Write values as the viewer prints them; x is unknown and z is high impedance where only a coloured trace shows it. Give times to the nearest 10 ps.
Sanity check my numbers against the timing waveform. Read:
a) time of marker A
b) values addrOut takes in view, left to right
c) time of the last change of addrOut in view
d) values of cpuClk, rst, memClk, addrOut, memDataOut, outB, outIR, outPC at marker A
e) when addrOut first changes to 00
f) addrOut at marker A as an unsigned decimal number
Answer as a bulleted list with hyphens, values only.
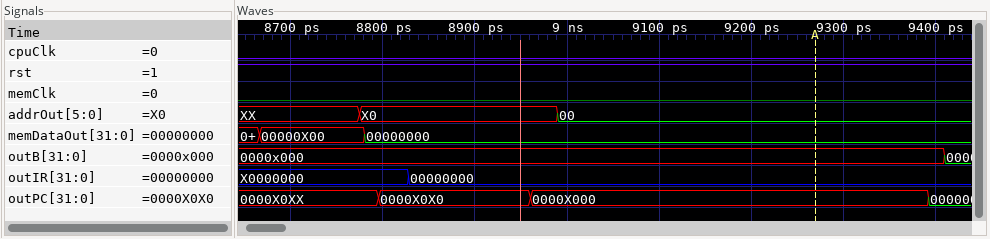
- 9270 ps
- XX, X0, 00
- 8990 ps
- cpuClk=0, rst=1, memClk=0, addrOut=00, memDataOut=00000000, outB=0000x000, outIR=00000000, outPC=0000X000
- 8990 ps
- 0
